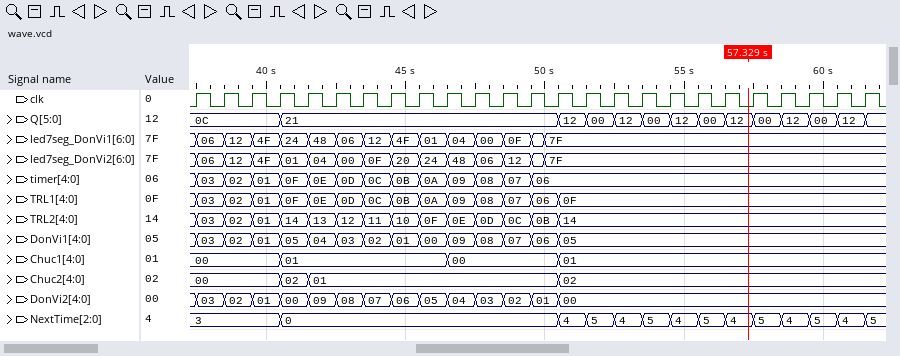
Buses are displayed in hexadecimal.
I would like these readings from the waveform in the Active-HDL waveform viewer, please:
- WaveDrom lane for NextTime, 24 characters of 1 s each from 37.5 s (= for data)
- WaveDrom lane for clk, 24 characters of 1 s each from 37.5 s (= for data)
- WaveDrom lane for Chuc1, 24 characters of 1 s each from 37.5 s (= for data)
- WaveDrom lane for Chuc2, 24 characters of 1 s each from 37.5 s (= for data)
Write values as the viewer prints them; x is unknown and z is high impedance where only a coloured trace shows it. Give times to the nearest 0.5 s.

{name: 'NextTime', wave: '=..=.........===========', data: '3 0 4 5 4 5 4 5 4 5 4 5 4'}
{name: 'clk', wave: 'p.......................'}
{name: 'Chuc1', wave: '=..=.....=...=..........', data: '00 01 00 01'}
{name: 'Chuc2', wave: '=..==........=..........', data: '00 02 01 02'}
